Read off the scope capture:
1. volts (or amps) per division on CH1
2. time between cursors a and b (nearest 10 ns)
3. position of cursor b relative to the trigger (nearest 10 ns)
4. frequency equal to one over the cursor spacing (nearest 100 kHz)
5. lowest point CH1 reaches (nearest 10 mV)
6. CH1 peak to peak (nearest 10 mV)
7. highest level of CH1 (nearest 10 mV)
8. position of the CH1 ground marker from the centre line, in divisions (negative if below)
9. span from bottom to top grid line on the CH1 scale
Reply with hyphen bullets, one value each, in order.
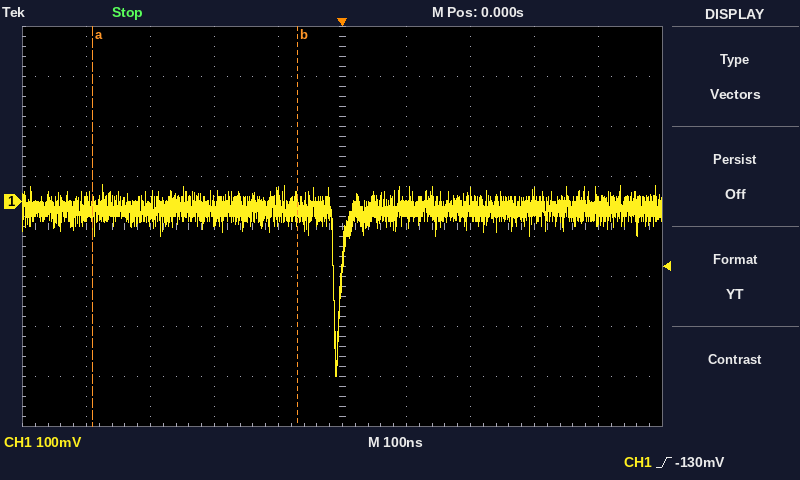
- 100 mV
- 320 ns
- -70 ns
- 3.1 MHz
- -350 mV
- 380 mV
- 30 mV
- +0.5 div
- 800 mV
